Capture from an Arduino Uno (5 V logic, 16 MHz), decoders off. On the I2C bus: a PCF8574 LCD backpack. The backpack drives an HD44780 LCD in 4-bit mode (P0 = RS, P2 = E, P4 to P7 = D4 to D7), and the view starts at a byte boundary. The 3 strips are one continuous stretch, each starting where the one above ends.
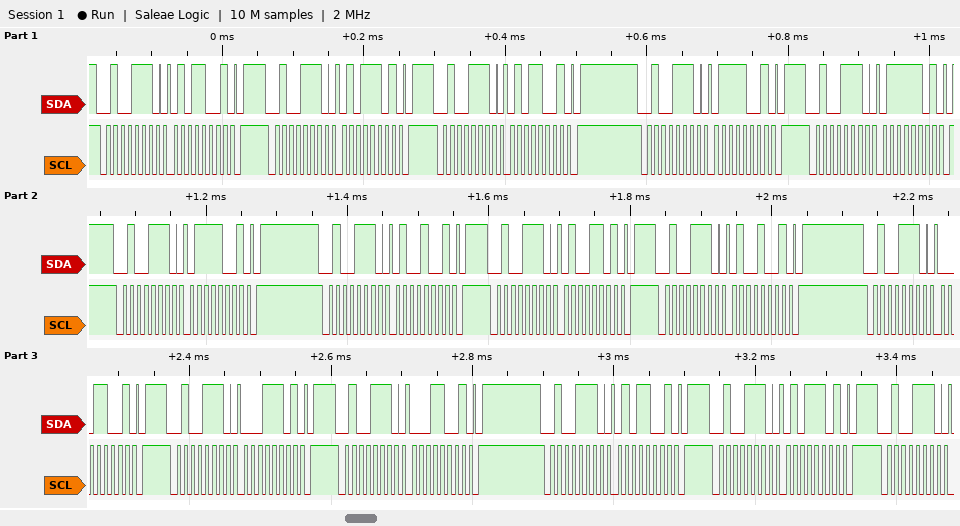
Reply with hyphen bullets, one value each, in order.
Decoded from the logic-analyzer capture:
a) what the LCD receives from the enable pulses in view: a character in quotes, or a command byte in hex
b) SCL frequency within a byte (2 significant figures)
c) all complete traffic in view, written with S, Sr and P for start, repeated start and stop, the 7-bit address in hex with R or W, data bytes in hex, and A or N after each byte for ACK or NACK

- 'W' 'A'
- 100 kHz
- S 27W A 59 A P S 27W A 5D A P S 27W A 59 A P S 27W A 79 A P S 27W A 7D A P S 27W A 79 A P S 27W A 49 A P S 27W A 4D A P S 27W A 49 A P S 27W A 19 A P S 27W A 1D A P S 27W A 19 A P S 27W A 59 A P S 27W A 5D A P S 27W A
